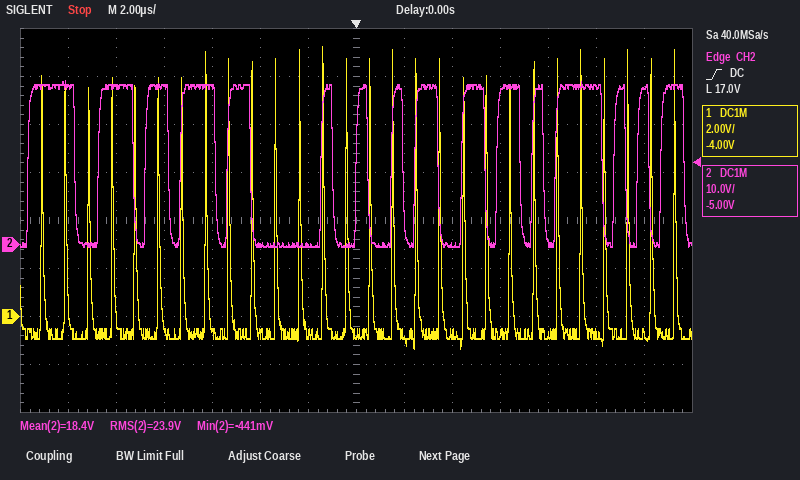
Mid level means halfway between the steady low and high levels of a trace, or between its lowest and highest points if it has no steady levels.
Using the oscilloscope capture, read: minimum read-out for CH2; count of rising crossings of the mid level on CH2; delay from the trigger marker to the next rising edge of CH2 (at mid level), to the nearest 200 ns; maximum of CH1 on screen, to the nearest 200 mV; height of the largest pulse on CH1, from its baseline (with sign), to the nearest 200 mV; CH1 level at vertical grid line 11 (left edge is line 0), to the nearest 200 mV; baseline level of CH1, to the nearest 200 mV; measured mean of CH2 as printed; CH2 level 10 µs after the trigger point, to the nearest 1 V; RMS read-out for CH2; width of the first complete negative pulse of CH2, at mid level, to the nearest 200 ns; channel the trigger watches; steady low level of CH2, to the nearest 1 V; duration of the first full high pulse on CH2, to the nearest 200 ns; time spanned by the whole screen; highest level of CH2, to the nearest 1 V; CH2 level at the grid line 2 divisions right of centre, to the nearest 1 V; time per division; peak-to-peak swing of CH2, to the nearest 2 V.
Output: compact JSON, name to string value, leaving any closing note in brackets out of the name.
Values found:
{"minimum read-out for CH2": "-441 mV", "count of rising crossings of the mid level on CH2": "16", "delay from the trigger marker to the next rising edge of CH2 (at mid level), to the nearest 200 ns": "1.4 µs", "maximum of CH1 on screen, to the nearest 200 mV": "11.2 V", "height of the largest pulse on CH1, from its baseline (with sign), to the nearest 200 mV": "+12.0 V", "CH1 level at vertical grid line 11 (left edge is line 0), to the nearest 200 mV": "-800 mV", "baseline level of CH1, to the nearest 200 mV": "-800 mV", "measured mean of CH2 as printed": "18.4 V", "CH2 level 10 µs after the trigger point, to the nearest 1 V": "33 V", "RMS read-out for CH2": "23.9 V", "width of the first complete negative pulse of CH2, at mid level, to the nearest 200 ns": "1.0 µs", "channel the trigger watches": "CH2", "steady low level of CH2, to the nearest 1 V": "0 V", "duration of the first full high pulse on CH2, to the nearest 200 ns": "2.0 µs", "time spanned by the whole screen": "28 µs", "highest level of CH2, to the nearest 1 V": "34 V", "CH2 level at the grid line 2 divisions right of centre, to the nearest 1 V": "0 V", "time per division": "2 µs", "peak-to-peak swing of CH2, to the nearest 2 V": "34 V"}
